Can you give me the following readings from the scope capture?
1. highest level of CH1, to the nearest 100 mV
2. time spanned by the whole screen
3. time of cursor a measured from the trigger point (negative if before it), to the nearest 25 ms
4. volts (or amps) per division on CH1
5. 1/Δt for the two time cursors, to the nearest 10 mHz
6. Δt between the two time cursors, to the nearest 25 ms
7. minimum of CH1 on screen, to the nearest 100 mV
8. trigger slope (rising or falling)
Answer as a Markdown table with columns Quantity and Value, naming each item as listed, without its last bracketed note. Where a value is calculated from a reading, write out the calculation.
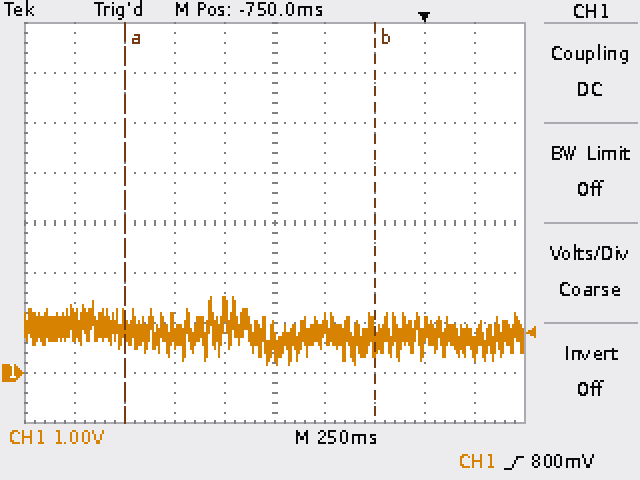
| Quantity | Value |
|---|---|
| highest level of CH1, to the nearest 100 mV | 1.5 V |
| time spanned by the whole screen | 2.5 s |
| time of cursor a measured from the trigger point (negative if before it), to the nearest 25 ms | -1.500 s |
| volts (or amps) per division on CH1 | 1 V |
| 1/Δt for the two time cursors, to the nearest 10 mHz | 1 / 1.250 s ≈ 800 mHz |
| Δt between the two time cursors, to the nearest 25 ms | 1.250 s |
| minimum of CH1 on screen, to the nearest 100 mV | 200 mV |
| trigger slope | rising |
